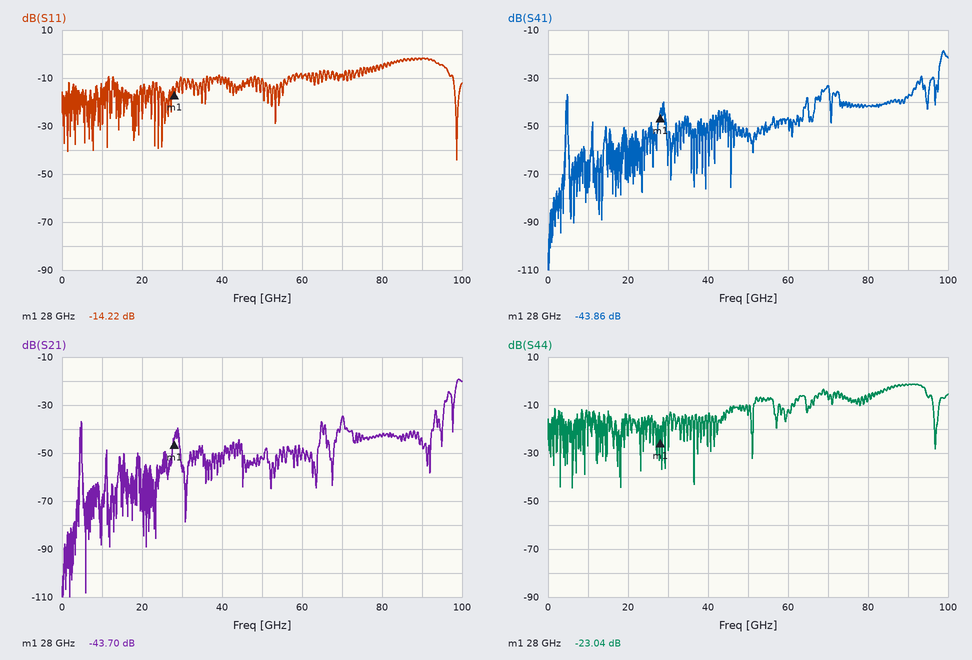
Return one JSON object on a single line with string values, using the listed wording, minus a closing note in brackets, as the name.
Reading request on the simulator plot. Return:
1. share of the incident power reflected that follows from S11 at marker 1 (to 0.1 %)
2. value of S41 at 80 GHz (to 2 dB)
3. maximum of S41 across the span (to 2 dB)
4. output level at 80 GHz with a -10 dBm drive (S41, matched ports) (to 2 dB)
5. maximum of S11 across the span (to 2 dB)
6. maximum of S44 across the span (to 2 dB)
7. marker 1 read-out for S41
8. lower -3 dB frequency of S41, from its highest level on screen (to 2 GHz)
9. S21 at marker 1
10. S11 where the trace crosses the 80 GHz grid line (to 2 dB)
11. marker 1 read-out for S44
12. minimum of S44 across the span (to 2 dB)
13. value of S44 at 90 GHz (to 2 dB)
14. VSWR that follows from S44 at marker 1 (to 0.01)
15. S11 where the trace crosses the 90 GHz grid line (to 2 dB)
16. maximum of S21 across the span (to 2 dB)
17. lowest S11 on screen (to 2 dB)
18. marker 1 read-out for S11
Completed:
{"share of the incident power reflected that follows from S11 at marker 1": "3.8 %", "value of S41 at 80 GHz": "-42 dB", "maximum of S41 across the span": "-18 dB", "output level at 80 GHz with a -10 dBm drive (S41, matched ports)": "-52 dBm", "maximum of S11 across the span": "-2 dB", "maximum of S44 across the span": "-2 dB", "marker 1 read-out for S41": "-43.86 dB", "lower -3 dB frequency of S41, from its highest level on screen": "98 GHz", "S21 at marker 1": "-43.70 dB", "S11 where the trace crosses the 80 GHz grid line": "-6 dB", "marker 1 read-out for S44": "-23.04 dB", "minimum of S44 across the span": "-44 dB", "value of S44 at 90 GHz": "-2 dB", "VSWR that follows from S44 at marker 1": "1.15", "S11 where the trace crosses the 90 GHz grid line": "-2 dB", "maximum of S21 across the span": "-20 dB", "lowest S11 on screen": "-44 dB", "marker 1 read-out for S11": "-14.22 dB"}
